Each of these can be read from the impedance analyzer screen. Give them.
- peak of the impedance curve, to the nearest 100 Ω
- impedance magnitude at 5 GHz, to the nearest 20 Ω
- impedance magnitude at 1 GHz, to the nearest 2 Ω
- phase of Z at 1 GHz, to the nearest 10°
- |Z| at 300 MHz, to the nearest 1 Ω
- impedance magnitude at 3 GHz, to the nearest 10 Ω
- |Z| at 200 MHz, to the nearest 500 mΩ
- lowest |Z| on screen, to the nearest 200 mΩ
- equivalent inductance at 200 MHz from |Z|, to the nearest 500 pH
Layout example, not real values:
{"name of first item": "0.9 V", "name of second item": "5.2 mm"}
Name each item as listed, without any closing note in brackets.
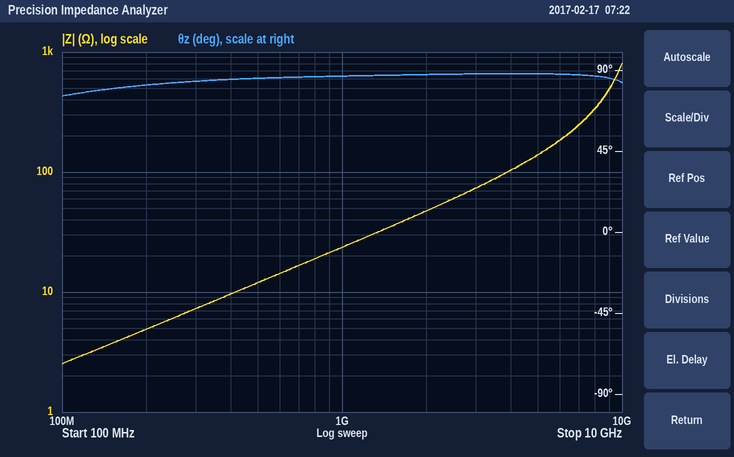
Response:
{"peak of the impedance curve, to the nearest 100 Ω": "800 Ω", "impedance magnitude at 5 GHz, to the nearest 20 Ω": "140 Ω", "impedance magnitude at 1 GHz, to the nearest 2 Ω": "24 Ω", "phase of Z at 1 GHz, to the nearest 10°": "90°", "|Z| at 300 MHz, to the nearest 1 Ω": "7 Ω", "impedance magnitude at 3 GHz, to the nearest 10 Ω": "70 Ω", "|Z| at 200 MHz, to the nearest 500 mΩ": "5.0 Ω", "lowest |Z| on screen, to the nearest 200 mΩ": "2.6 Ω", "equivalent inductance at 200 MHz from |Z|, to the nearest 500 pH": "4.0 nH"}
